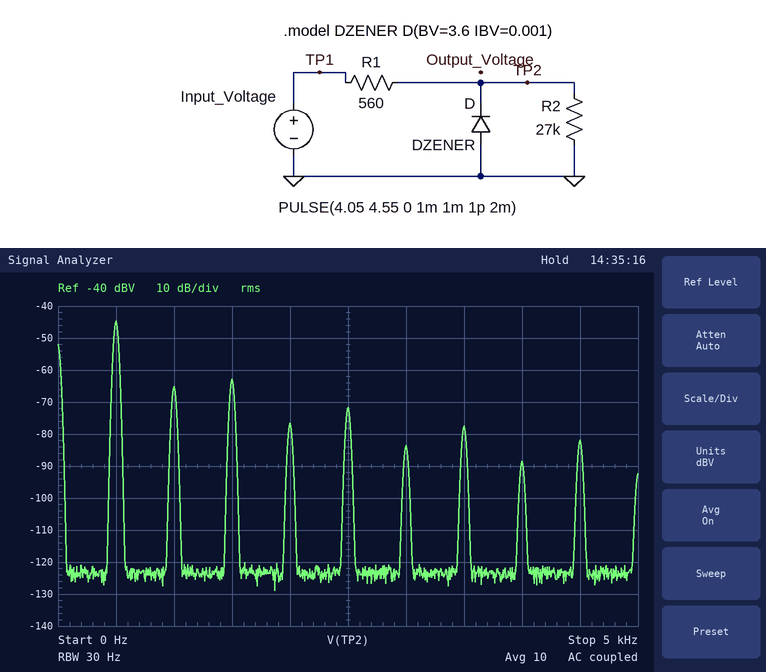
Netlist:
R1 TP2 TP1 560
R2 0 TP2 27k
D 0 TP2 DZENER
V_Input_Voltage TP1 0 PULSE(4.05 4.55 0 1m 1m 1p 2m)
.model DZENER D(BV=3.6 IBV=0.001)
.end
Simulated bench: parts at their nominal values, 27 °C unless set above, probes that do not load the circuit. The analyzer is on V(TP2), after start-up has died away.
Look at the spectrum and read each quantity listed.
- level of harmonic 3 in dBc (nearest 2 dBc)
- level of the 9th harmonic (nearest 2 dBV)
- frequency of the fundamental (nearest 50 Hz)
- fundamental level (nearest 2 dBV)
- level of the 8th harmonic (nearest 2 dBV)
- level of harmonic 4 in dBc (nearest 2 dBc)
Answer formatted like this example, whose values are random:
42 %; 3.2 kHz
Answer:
-18 dBc; -82 dBV; 500 Hz; -44 dBV; -88 dBV; -32 dBc
